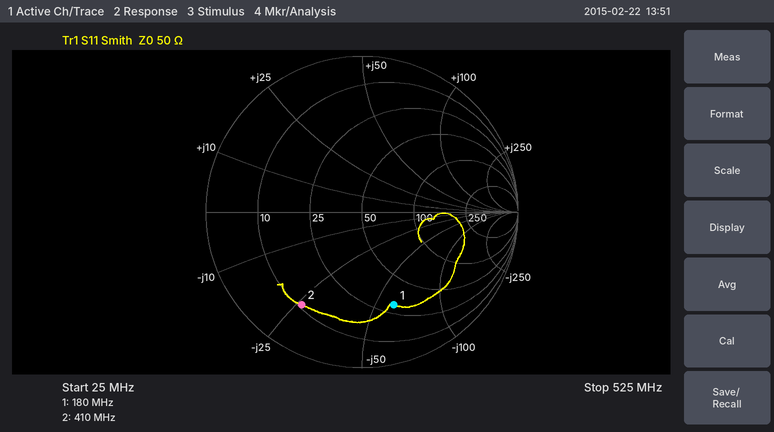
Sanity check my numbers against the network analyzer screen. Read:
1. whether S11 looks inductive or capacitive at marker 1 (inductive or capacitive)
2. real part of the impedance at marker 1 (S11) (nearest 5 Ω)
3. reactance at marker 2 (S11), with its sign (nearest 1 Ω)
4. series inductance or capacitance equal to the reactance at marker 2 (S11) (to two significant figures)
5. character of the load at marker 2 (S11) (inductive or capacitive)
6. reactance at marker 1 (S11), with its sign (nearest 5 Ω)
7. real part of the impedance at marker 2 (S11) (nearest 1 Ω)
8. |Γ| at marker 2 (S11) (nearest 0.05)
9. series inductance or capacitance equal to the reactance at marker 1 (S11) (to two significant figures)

capacitive
30 Ω
-26 Ω
15 pF
capacitive
-60 Ω
11 Ω
0.70
15 pF
